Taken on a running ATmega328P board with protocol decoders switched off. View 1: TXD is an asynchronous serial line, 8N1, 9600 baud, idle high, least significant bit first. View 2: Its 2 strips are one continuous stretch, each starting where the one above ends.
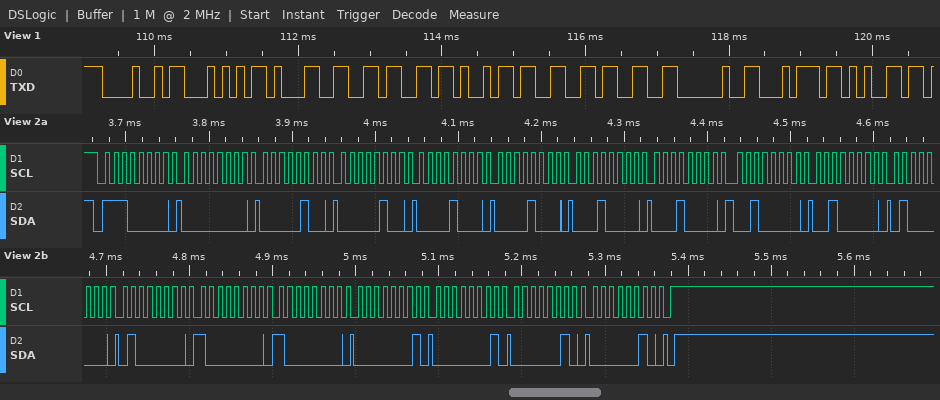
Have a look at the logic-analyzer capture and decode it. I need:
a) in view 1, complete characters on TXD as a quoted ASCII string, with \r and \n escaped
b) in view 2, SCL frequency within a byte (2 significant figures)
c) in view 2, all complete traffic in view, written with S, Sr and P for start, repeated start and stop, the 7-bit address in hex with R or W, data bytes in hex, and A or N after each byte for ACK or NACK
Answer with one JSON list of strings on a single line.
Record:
["\"HT16K33 te\"", "100 kHz", "S 70W A 00 A 04 A 04 A 08 A 08 A 10 A 10 A 20 A 20 A 40 A 40 A 80 A 80 A 01 A 01 A 02 A 02 A P"]
